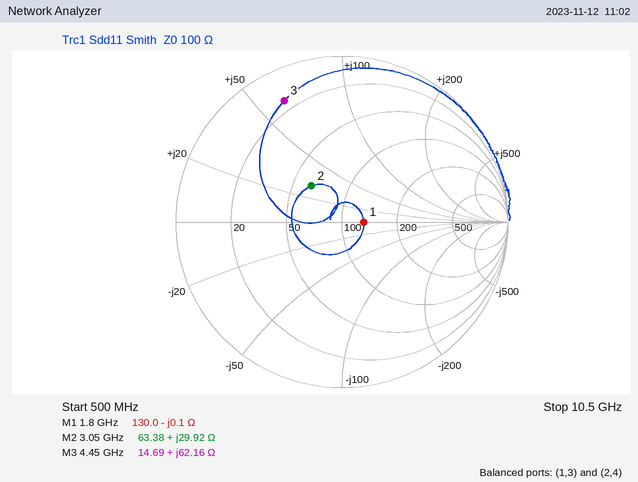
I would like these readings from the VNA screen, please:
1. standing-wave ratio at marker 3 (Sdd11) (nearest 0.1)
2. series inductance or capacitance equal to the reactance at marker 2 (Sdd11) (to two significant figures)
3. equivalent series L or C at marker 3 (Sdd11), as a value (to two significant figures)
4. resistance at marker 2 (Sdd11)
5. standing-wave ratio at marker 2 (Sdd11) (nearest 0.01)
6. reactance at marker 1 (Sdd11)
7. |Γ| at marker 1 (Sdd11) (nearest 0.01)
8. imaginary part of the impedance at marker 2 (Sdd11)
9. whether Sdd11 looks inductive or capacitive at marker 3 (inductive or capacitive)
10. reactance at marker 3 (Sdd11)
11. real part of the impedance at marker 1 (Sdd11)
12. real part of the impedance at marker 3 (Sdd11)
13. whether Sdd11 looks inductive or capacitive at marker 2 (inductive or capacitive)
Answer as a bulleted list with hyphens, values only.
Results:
- 9.5
- 1.6 nH
- 2.2 nH
- 63.38 Ω
- 1.80
- -0.1 Ω
- 0.13
- +29.92 Ω
- inductive
- +62.16 Ω
- 130.0 Ω
- 14.69 Ω
- inductive
